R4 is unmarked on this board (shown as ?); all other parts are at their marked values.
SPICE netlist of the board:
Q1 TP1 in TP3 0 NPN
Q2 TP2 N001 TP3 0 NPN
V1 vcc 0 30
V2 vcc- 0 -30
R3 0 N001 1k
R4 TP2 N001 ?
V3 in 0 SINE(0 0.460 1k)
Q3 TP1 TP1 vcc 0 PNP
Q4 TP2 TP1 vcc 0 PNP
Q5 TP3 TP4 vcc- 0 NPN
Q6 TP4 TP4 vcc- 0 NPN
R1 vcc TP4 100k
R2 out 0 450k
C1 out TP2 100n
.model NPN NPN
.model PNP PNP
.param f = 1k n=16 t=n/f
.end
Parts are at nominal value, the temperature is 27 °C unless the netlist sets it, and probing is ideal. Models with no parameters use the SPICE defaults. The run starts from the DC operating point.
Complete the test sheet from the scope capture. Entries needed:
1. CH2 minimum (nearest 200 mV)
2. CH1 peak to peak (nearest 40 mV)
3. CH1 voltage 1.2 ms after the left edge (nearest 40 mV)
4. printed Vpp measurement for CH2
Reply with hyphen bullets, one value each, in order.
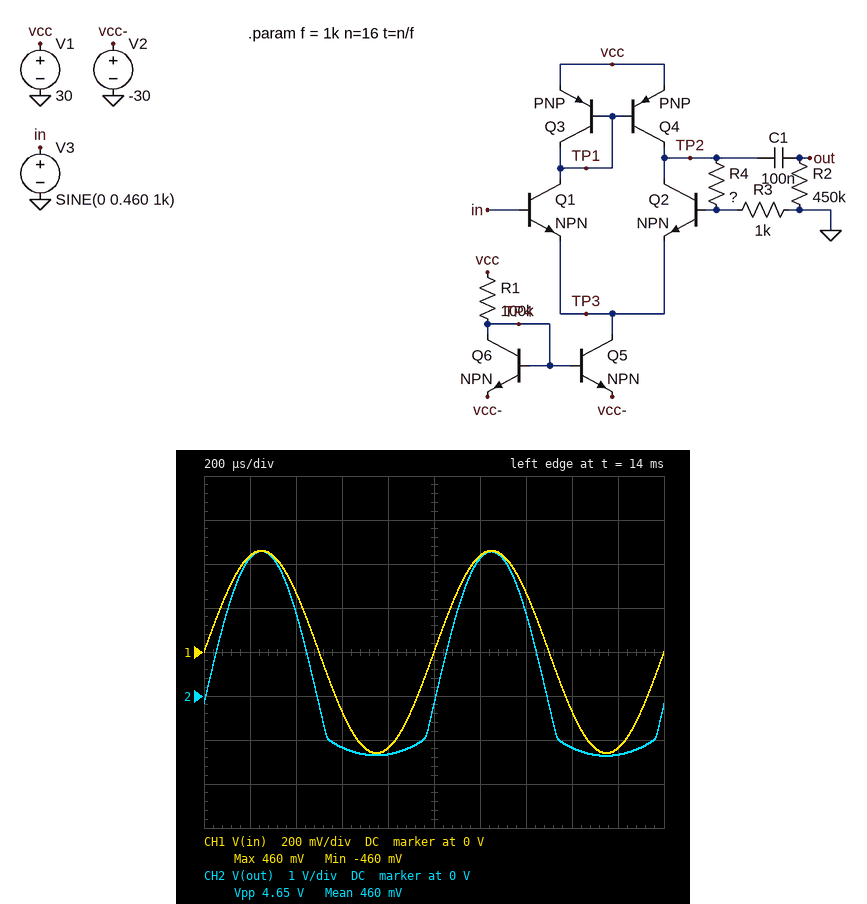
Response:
- -1.4 V
- 920 mV
- 440 mV
- 4.65 V
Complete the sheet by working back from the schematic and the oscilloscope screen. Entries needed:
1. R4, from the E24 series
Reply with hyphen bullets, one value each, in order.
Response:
- 7.5 kΩ
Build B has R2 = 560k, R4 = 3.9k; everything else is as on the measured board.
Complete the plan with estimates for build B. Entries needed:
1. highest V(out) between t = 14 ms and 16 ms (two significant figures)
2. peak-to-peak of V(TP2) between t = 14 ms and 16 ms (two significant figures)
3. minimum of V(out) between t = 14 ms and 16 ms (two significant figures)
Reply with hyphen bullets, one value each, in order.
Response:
- 2.0 V
- 3.2 V
- -1.2 V
